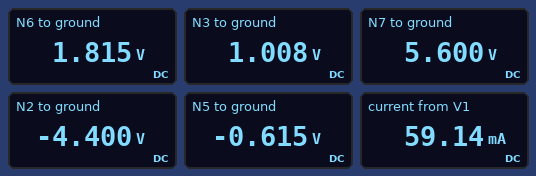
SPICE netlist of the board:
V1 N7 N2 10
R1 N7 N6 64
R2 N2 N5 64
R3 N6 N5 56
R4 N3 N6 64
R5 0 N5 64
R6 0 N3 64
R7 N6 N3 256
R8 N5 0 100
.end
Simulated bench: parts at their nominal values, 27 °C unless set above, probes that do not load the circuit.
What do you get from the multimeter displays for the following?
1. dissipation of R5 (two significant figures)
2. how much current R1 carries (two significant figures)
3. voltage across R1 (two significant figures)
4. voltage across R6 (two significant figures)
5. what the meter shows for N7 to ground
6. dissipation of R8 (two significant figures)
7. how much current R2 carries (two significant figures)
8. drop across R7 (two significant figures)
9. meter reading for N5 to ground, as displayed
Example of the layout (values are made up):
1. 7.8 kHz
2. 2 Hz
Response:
1. 5.9 mW
2. 59 mA
3. 3.8 V
4. 1.0 V
5. 5.600 V
6. 3.8 mW
7. 59 mA
8. 810 mV
9. -0.615 V
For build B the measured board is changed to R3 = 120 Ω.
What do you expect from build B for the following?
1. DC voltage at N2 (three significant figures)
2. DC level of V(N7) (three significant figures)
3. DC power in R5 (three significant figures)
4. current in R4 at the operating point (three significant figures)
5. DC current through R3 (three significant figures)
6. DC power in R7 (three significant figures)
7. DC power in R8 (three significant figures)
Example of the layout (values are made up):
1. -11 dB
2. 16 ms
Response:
1. -4.15 V
2. 5.85 V
3. 11.9 mW
4. 17.9 mA
5. 28.8 mA
6. 5.13 mW
7. 7.63 mW
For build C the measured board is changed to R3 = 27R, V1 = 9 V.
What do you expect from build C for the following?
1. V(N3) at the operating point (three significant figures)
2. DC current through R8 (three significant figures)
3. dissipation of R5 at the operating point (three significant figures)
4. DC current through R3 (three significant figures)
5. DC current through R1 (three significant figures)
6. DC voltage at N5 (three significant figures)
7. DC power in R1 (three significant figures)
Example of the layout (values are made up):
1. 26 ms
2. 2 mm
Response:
1. 568 mV
2. 3.47 mA
3. 1.88 mW
4. 50.7 mA
5. 59.6 mA
6. -347 mV
7. 227 mW
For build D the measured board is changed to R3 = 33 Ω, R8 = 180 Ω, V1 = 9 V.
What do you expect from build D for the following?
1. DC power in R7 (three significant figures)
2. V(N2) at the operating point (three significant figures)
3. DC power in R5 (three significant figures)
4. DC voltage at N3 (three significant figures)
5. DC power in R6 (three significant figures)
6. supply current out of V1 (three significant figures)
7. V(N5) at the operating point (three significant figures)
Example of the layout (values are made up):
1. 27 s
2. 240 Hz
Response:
1. 979 µW
2. -4.17 V
3. 3.33 mW
4. 626 mV
5. 6.12 mW
6. 57.9 mA
7. -462 mV
